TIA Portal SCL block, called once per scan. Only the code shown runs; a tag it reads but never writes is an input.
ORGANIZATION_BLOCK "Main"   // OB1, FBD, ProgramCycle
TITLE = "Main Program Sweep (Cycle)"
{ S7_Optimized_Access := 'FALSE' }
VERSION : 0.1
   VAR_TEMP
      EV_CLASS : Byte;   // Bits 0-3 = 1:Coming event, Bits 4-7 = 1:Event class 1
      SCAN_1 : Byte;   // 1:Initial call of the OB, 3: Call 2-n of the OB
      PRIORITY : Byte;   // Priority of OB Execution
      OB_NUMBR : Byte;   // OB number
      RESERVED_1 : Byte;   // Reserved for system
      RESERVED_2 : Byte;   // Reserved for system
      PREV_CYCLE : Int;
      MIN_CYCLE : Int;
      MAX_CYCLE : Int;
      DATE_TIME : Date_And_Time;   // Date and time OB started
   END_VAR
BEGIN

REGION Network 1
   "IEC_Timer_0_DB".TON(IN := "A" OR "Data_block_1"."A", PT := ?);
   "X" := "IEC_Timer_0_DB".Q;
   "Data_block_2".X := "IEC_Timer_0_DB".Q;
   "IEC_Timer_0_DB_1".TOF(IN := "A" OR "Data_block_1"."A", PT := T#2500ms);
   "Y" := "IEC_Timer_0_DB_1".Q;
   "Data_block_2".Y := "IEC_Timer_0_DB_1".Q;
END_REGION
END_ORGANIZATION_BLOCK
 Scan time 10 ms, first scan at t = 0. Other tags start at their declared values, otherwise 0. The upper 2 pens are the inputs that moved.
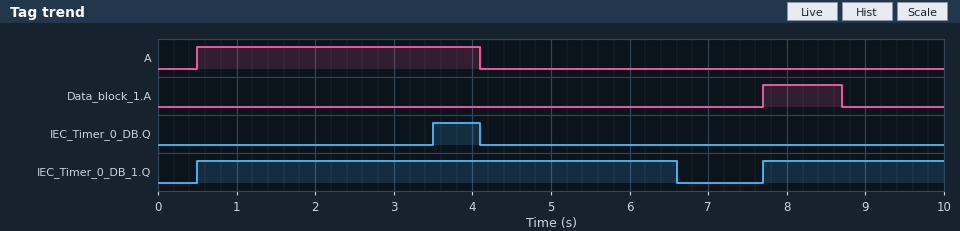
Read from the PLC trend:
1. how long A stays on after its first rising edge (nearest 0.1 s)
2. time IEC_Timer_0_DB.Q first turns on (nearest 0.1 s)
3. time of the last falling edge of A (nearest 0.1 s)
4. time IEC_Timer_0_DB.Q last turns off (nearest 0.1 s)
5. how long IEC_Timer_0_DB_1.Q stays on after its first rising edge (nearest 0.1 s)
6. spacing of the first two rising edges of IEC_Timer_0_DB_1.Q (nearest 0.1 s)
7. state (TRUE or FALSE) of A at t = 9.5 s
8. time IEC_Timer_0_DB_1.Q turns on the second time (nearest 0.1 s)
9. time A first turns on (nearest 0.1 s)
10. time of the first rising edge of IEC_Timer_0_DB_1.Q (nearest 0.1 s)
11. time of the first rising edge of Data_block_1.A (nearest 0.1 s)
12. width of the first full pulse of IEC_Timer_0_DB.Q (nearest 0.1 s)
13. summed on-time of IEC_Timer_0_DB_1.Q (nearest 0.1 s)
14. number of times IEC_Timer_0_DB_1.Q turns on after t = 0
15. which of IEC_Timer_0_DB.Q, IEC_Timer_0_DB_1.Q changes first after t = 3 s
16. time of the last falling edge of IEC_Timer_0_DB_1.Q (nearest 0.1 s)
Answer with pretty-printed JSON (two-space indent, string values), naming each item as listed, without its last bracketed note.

{
  "how long A stays on after its first rising edge": "3.6 s",
  "time IEC_Timer_0_DB.Q first turns on": "3.5 s",
  "time of the last falling edge of A": "4.1 s",
  "time IEC_Timer_0_DB.Q last turns off": "4.1 s",
  "how long IEC_Timer_0_DB_1.Q stays on after its first rising edge": "6.1 s",
  "spacing of the first two rising edges of IEC_Timer_0_DB_1.Q": "7.2 s",
  "state (TRUE or FALSE) of A at t = 9.5 s": "FALSE",
  "time IEC_Timer_0_DB_1.Q turns on the second time": "7.7 s",
  "time A first turns on": "0.5 s",
  "time of the first rising edge of IEC_Timer_0_DB_1.Q": "0.5 s",
  "time of the first rising edge of Data_block_1.A": "7.7 s",
  "width of the first full pulse of IEC_Timer_0_DB.Q": "0.6 s",
  "summed on-time of IEC_Timer_0_DB_1.Q": "8.4 s",
  "number of times IEC_Timer_0_DB_1.Q turns on after t = 0": "2",
  "which of IEC_Timer_0_DB.Q, IEC_Timer_0_DB_1.Q changes first after t = 3 s": "IEC_Timer_0_DB.Q",
  "time of the last falling edge of IEC_Timer_0_DB_1.Q": "6.6 s"
}
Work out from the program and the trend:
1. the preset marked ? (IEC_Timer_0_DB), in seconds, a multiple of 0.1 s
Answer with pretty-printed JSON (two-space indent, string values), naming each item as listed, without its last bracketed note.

{
  "the preset marked ? (IEC_Timer_0_DB), in seconds, a multiple of 0.1 s": "3.0 s"
}
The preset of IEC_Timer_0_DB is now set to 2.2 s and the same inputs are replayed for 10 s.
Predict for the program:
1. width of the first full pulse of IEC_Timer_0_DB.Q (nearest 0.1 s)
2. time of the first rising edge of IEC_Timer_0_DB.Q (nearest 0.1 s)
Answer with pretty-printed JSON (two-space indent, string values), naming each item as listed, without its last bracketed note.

{
  "width of the first full pulse of IEC_Timer_0_DB.Q": "1.4 s",
  "time of the first rising edge of IEC_Timer_0_DB.Q": "2.7 s"
}
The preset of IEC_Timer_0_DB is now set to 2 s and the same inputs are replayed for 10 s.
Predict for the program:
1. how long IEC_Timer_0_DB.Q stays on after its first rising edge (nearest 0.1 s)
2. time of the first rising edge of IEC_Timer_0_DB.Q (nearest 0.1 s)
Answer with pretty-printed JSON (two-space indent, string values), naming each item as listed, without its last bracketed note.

{
  "how long IEC_Timer_0_DB.Q stays on after its first rising edge": "1.6 s",
  "time of the first rising edge of IEC_Timer_0_DB.Q": "2.5 s"
}
